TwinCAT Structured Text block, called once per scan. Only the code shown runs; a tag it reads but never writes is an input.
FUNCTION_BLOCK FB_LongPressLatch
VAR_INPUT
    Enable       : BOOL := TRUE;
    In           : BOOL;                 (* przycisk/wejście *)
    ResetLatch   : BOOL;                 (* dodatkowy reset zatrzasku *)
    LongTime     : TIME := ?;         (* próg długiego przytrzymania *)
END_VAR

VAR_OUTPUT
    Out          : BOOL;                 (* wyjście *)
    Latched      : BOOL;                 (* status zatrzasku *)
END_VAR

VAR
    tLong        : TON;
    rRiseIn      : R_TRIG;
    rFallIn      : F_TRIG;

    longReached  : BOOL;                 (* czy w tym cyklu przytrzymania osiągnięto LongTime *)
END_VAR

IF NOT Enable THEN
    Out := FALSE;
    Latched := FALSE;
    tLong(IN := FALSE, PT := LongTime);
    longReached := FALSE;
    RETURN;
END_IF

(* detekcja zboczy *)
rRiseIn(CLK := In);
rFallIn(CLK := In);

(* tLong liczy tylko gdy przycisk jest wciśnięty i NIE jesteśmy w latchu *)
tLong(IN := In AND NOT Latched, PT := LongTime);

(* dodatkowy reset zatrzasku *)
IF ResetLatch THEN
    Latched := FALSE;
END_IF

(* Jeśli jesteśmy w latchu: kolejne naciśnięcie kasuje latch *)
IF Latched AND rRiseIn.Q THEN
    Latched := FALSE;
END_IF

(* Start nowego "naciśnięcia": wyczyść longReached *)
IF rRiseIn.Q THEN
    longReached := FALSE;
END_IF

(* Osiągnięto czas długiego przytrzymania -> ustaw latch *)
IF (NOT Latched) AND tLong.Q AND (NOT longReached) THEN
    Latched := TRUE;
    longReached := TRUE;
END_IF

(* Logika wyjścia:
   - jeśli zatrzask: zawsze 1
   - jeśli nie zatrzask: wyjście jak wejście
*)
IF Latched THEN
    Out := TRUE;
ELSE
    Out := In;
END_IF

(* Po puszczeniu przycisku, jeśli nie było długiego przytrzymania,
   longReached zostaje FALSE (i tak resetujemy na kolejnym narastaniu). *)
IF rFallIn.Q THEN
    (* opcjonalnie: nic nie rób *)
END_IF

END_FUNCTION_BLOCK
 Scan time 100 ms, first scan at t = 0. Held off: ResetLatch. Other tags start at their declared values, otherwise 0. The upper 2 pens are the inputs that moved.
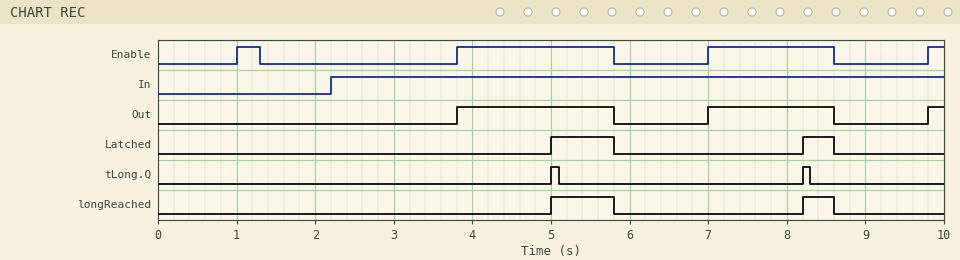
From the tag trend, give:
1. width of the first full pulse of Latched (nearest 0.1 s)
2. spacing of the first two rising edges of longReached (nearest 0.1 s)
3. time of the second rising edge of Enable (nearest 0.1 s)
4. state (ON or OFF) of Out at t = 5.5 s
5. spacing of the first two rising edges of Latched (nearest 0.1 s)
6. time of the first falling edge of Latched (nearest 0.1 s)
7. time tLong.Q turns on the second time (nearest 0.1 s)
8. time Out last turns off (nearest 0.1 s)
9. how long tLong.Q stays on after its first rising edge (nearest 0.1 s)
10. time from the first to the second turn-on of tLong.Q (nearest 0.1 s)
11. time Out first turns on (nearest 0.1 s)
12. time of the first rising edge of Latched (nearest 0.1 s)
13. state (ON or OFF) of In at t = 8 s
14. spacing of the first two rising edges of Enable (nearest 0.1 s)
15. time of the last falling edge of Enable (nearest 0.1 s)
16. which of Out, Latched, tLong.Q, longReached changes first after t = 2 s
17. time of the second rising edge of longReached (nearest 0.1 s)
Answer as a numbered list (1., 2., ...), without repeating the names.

1. 0.8 s
2. 3.2 s
3. 3.8 s
4. ON
5. 3.2 s
6. 5.8 s
7. 8.2 s
8. 8.6 s
9. 0.1 s
10. 3.2 s
11. 3.8 s
12. 5.0 s
13. ON
14. 2.8 s
15. 8.6 s
16. Out
17. 8.2 s
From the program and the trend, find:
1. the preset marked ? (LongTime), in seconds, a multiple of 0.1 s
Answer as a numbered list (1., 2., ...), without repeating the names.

1. 1.2 s
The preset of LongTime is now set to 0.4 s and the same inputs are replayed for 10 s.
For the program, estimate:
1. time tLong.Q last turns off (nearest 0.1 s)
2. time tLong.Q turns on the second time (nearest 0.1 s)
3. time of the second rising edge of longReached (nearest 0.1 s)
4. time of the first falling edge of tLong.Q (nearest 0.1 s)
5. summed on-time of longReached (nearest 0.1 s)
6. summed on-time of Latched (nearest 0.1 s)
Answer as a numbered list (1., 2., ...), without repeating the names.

1. 7.5 s
2. 7.4 s
3. 7.4 s
4. 4.3 s
5. 2.8 s
6. 2.8 s
